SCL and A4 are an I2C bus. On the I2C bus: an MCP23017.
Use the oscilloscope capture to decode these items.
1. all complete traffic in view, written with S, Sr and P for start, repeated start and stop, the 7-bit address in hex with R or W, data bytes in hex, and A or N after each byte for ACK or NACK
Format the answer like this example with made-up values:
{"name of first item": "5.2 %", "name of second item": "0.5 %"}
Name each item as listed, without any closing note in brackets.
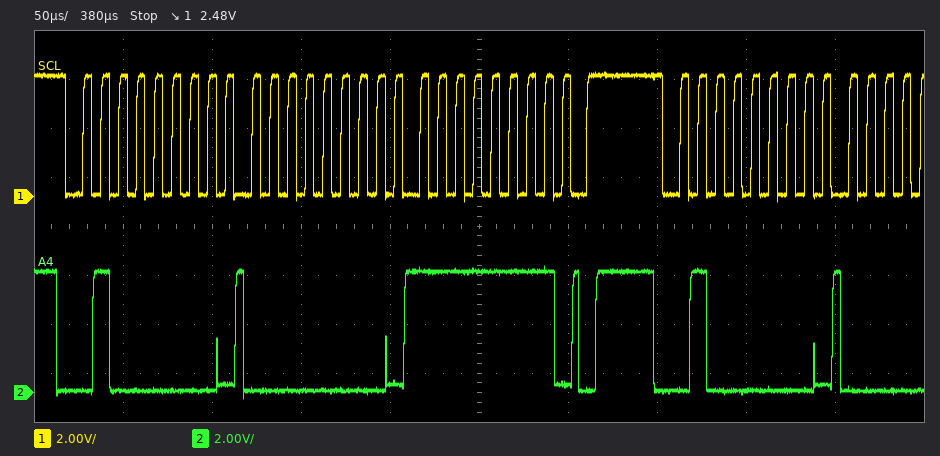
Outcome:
{"all complete traffic in view, written with S, Sr and P for start, repeated start and stop, the 7-bit address in hex with R or W, data bytes in hex, and A or N after each byte for ACK or NACK": "S 20W A 00 A FF A P S 20W A"}
